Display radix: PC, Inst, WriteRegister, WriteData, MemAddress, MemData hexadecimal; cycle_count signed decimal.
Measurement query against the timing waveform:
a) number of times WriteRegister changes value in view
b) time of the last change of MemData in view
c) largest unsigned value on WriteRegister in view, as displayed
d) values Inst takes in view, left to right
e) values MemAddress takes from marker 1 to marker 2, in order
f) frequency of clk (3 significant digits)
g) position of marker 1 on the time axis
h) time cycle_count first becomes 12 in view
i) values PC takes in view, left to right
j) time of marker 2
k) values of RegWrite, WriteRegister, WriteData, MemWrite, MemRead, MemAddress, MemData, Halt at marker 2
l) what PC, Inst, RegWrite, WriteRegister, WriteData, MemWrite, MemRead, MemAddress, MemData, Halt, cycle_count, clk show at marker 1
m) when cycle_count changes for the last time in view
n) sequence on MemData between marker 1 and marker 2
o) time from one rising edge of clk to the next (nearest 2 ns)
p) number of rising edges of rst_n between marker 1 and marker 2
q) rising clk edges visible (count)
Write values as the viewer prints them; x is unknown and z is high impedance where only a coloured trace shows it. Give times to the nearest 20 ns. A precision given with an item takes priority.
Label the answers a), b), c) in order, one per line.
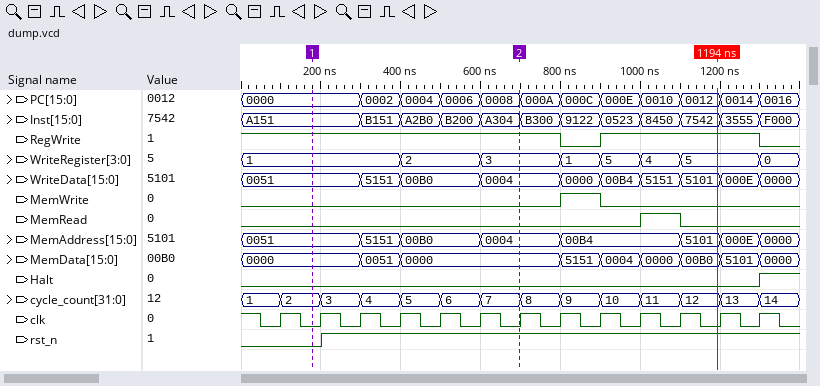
a) 7
b) 1300 ns
c) 5
d) A151, B151, A2B0, B200, A304, B300, 9122, 0523, 8450, 7542, 3555, F000
e) 0051, 5151, 00B0, 0004
f) 10.0 MHz
g) 180 ns
h) 1100 ns
i) 0000, 0002, 0004, 0006, 0008, 000A, 000C, 000E, 0010, 0012, 0014, 0016
j) 700 ns
k) RegWrite=1, WriteRegister=3, WriteData=0004, MemWrite=0, MemRead=0, MemAddress=0004, MemData=0000, Halt=0
l) PC=0000, Inst=A151, RegWrite=1, WriteRegister=1, WriteData=0051, MemWrite=0, MemRead=0, MemAddress=0051, MemData=0000, Halt=0, cycle_count=2, clk=0
m) 1300 ns
n) 0000, 0051, 0000
o) 100 ns
p) 1
q) 13
